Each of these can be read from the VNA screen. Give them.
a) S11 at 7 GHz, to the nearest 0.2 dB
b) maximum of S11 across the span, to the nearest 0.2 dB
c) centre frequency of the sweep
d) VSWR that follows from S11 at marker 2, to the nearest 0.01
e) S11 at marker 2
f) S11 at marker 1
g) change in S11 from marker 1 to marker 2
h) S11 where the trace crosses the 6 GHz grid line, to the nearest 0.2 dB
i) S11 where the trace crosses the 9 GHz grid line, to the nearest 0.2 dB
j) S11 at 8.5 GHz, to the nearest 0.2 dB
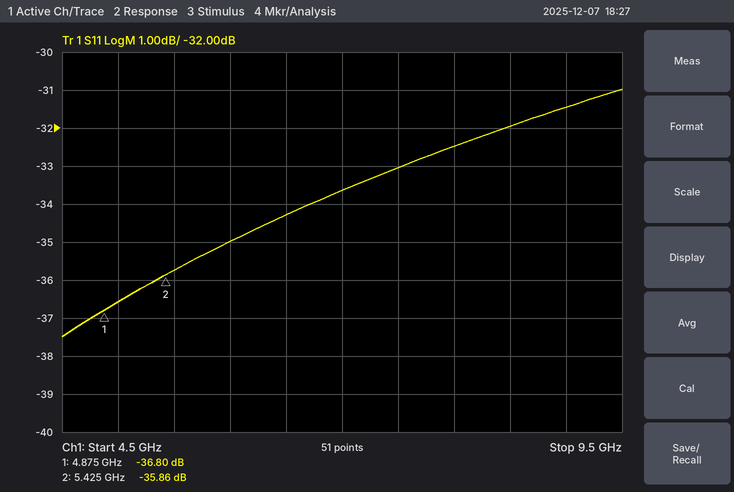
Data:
-33.6 dB
-31.0 dB
7 GHz
1.03
-35.86 dB
-36.80 dB
0.94 dB
-35.0 dB
-31.4 dB
-32.0 dB
